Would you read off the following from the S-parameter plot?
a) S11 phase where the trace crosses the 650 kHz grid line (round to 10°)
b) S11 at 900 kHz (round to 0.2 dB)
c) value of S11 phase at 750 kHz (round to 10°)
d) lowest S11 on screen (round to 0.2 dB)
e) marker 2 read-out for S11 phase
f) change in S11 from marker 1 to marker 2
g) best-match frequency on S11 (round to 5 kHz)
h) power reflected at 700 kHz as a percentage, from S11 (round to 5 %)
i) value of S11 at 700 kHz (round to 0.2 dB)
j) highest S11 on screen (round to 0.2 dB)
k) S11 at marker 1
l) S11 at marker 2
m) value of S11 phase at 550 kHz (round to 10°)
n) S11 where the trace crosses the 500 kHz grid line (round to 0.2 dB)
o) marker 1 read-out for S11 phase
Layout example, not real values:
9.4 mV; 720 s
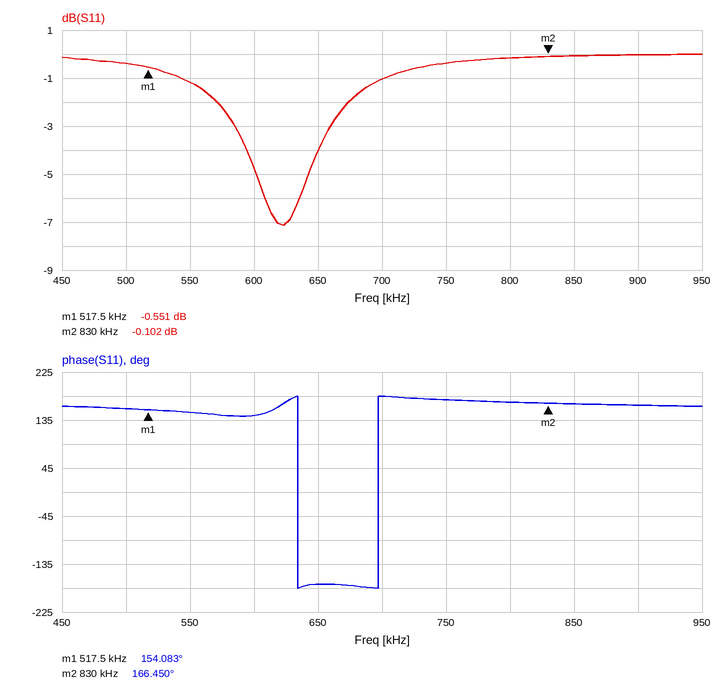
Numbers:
-170°; 0.0 dB; 170°; -7.2 dB; 166.450°; 0.449 dB; 625 kHz; 80 %; -1.0 dB; 0.0 dB; -0.551 dB; -0.102 dB; 150°; -0.4 dB; 154.083°
